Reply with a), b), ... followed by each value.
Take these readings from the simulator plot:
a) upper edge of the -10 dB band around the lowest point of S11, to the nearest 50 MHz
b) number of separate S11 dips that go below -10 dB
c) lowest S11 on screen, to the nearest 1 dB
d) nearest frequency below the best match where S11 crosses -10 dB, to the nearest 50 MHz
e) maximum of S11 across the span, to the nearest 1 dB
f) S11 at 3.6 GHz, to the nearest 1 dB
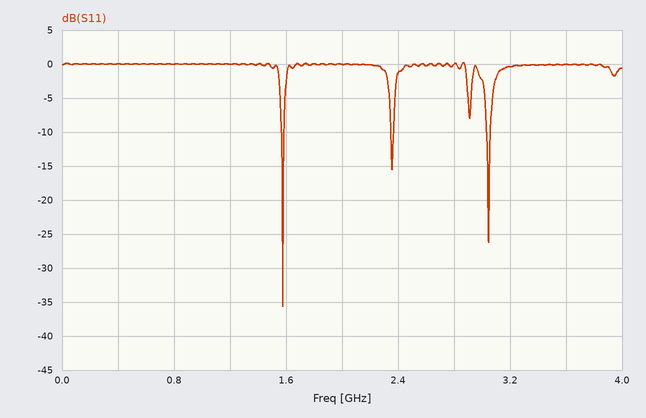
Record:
a) 1.60 GHz
b) 3
c) -36 dB
d) 1.55 GHz
e) 0 dB
f) 0 dB
